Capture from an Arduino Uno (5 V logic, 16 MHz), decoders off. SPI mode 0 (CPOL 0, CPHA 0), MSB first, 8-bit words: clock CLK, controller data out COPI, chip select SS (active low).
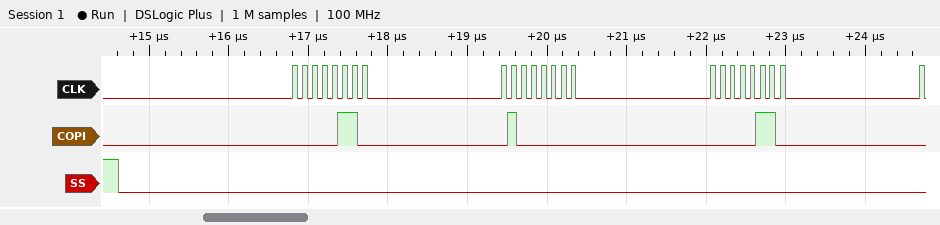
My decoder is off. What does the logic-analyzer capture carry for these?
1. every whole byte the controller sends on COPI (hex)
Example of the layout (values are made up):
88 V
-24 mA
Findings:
06 40 06
